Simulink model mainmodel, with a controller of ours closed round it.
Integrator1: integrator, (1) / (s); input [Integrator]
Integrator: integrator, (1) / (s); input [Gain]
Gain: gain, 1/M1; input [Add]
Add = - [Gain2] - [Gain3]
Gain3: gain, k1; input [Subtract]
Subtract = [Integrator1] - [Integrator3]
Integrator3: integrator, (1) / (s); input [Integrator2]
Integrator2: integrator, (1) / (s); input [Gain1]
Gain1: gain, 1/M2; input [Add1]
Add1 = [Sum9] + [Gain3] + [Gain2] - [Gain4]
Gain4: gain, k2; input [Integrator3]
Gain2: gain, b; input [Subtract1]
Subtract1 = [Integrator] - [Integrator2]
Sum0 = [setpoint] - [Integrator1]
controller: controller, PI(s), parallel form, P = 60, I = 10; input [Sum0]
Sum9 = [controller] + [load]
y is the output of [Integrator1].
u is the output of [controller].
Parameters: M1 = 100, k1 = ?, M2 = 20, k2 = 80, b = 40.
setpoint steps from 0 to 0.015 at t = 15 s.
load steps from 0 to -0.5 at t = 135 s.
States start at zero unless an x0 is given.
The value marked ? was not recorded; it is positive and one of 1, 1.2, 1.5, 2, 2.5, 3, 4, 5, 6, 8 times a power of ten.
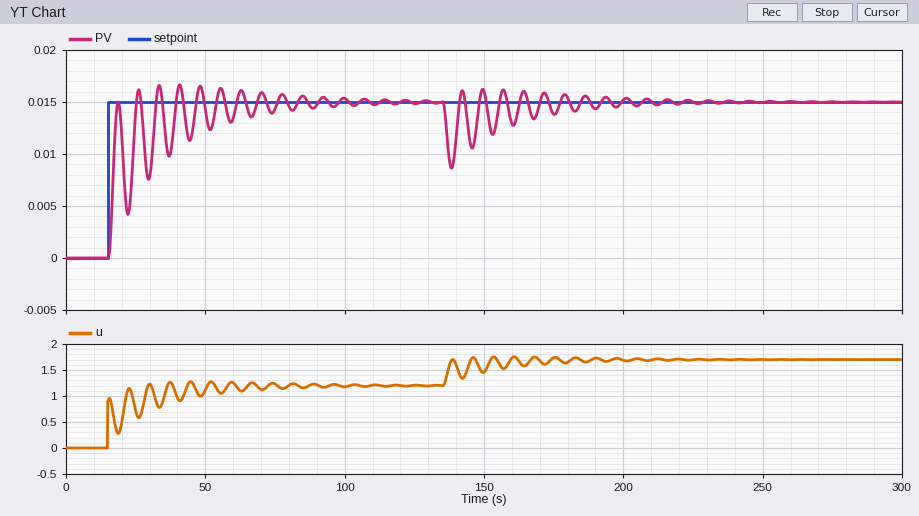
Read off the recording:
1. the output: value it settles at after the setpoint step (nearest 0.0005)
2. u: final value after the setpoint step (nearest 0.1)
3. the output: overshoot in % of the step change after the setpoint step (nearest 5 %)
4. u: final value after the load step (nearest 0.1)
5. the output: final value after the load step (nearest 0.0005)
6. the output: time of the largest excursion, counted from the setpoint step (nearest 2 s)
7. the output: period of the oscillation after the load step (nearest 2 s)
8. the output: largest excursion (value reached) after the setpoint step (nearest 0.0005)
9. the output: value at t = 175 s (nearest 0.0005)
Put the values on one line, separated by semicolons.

0.0150; 1.2; 10 %; 1.7; 0.0150; 26 s; 8 s; 0.0165; 0.0140
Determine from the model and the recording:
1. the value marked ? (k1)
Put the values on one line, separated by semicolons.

80
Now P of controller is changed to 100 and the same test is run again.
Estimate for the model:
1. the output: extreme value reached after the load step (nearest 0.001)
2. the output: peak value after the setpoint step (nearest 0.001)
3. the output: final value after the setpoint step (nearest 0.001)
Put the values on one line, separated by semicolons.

0.010; 0.018; 0.015
